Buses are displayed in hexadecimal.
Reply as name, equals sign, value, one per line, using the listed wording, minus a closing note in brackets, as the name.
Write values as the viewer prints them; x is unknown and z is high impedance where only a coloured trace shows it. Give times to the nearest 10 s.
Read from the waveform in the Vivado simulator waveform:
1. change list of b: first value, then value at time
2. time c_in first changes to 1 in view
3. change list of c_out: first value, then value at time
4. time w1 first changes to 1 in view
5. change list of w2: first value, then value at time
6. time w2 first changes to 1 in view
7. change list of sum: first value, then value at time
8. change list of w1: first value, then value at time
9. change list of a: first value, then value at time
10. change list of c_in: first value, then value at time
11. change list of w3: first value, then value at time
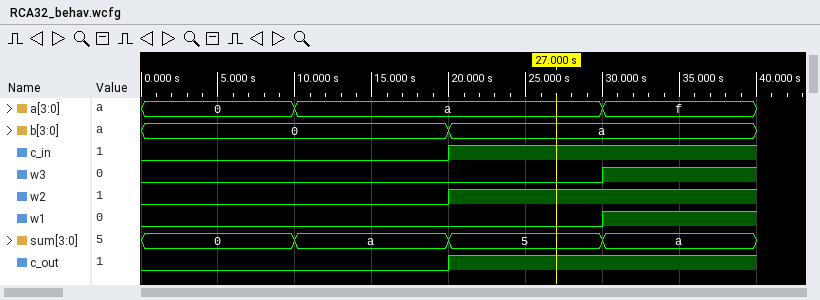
change list of b: first value, then value at time = 0, a at 20 s
time c_in first changes to 1 in view = 20 s
change list of c_out: first value, then value at time = 0, 1 at 20 s
time w1 first changes to 1 in view = 30 s
change list of w2: first value, then value at time = 0, 1 at 20 s
time w2 first changes to 1 in view = 20 s
change list of sum: first value, then value at time = 0, a at 10 s, 5 at 20 s, a at 30 s
change list of w1: first value, then value at time = 0, 1 at 30 s
change list of a: first value, then value at time = 0, a at 10 s, f at 30 s
change list of c_in: first value, then value at time = 0, 1 at 20 s
change list of w3: first value, then value at time = 0, 1 at 30 s
